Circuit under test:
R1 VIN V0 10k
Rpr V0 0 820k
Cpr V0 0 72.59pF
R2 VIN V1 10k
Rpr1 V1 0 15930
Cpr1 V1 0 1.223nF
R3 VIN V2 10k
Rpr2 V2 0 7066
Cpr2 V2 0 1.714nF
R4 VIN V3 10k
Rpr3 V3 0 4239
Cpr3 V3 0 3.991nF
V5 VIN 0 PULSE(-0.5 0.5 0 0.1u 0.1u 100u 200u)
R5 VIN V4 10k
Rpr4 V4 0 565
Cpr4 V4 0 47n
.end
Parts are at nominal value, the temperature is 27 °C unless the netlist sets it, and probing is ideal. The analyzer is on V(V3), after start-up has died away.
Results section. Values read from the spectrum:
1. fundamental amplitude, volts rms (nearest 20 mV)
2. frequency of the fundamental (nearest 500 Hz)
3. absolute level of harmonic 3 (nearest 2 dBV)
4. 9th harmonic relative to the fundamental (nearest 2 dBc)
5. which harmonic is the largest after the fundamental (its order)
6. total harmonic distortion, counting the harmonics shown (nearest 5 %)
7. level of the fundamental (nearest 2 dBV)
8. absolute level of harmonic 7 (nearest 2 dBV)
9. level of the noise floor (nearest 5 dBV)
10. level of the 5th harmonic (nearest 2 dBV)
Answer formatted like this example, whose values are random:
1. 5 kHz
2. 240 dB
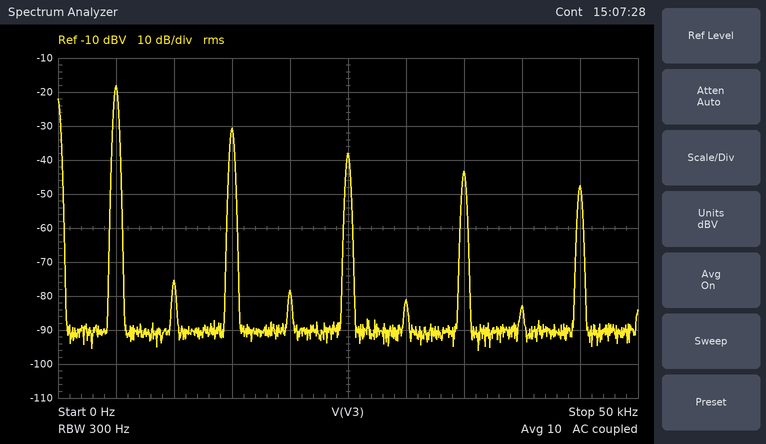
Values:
1. 120 mV
2. 5.0 kHz
3. -30 dBV
4. -30 dBc
5. 3
6. 25 %
7. -18 dBV
8. -44 dBV
9. -90 dBV
10. -38 dBV
